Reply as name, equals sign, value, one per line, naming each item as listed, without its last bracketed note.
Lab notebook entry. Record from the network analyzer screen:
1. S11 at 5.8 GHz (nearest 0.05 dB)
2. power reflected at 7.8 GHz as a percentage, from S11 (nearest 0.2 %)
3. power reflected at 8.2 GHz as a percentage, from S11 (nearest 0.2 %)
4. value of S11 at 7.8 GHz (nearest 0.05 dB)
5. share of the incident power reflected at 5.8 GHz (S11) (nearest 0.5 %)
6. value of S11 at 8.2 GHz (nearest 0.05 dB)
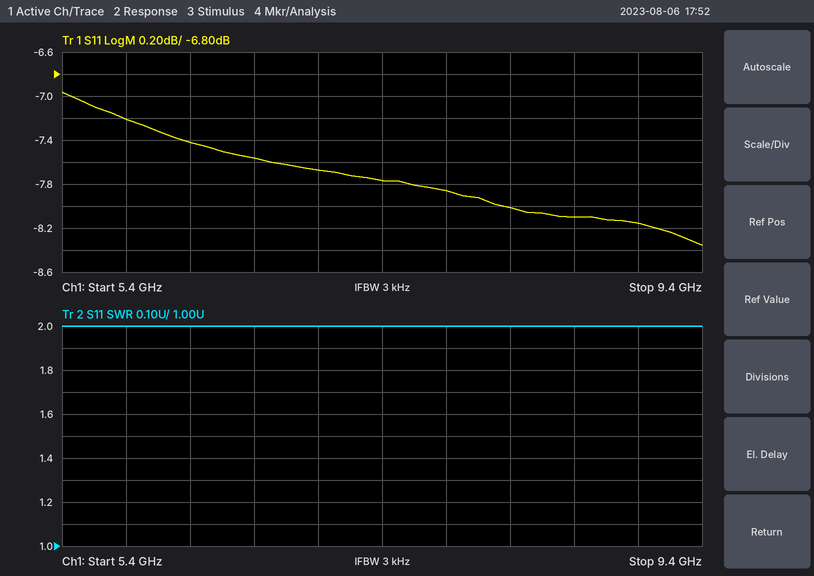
S11 at 5.8 GHz = -7.20 dB
power reflected at 7.8 GHz as a percentage, from S11 = 16.4 %
power reflected at 8.2 GHz as a percentage, from S11 = 15.8 %
value of S11 at 7.8 GHz = -7.85 dB
share of the incident power reflected at 5.8 GHz (S11) = 19.0 %
value of S11 at 8.2 GHz = -8.00 dB
